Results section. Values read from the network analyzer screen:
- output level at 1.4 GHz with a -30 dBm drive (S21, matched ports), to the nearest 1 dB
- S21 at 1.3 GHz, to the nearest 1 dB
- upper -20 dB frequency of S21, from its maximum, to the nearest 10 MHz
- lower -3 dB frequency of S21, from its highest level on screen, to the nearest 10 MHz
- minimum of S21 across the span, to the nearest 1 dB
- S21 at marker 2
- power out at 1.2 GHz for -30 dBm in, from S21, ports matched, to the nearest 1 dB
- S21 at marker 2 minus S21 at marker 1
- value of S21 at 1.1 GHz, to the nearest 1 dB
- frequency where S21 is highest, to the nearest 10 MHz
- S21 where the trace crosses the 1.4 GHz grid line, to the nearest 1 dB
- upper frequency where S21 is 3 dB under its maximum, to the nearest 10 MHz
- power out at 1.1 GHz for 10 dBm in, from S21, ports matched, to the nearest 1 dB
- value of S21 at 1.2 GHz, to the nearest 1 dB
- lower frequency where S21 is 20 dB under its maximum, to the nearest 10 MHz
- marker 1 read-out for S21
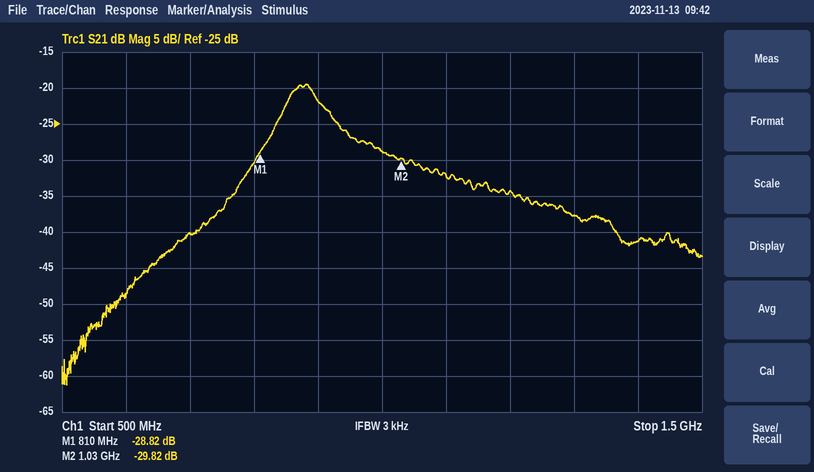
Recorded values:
-71 dBm
-38 dB
1.36 GHz
850 MHz
-61 dB
-29.82 dB
-64 dBm
-1.00 dB
-32 dB
880 MHz
-41 dB
910 MHz
-22 dBm
-34 dB
720 MHz
-28.82 dB
